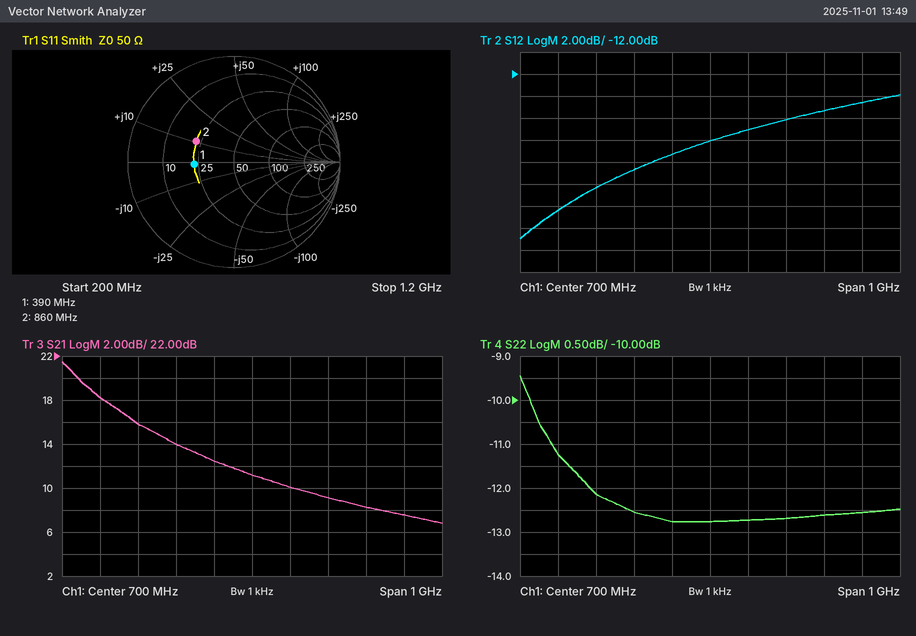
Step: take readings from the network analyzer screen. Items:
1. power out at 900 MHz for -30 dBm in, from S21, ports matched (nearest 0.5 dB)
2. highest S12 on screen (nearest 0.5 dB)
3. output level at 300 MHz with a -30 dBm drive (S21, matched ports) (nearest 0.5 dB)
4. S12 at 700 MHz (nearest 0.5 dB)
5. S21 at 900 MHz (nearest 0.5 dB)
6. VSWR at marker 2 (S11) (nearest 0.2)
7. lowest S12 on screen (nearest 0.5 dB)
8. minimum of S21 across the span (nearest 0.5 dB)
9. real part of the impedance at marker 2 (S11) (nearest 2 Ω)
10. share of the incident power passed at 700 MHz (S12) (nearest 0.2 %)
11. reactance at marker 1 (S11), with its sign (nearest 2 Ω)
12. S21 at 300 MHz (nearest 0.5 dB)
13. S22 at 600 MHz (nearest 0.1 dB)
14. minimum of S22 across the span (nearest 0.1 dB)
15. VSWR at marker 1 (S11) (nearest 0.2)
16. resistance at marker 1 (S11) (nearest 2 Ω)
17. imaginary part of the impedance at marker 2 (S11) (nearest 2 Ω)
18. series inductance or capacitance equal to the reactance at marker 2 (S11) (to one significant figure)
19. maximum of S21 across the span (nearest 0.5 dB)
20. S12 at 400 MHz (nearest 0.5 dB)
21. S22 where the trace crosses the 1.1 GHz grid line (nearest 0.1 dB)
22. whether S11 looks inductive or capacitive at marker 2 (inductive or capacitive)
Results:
-21.0 dBm
-14.0 dB
-12.0 dBm
-18.0 dB
9.0 dB
2.4
-27.0 dB
7.0 dB
22 Ω
1.6 %
-2 Ω
18.0 dB
-12.8 dB
-12.8 dB
2.2
22 Ω
+10 Ω
2 nH
21.5 dB
-22.5 dB
-12.6 dB
inductive
